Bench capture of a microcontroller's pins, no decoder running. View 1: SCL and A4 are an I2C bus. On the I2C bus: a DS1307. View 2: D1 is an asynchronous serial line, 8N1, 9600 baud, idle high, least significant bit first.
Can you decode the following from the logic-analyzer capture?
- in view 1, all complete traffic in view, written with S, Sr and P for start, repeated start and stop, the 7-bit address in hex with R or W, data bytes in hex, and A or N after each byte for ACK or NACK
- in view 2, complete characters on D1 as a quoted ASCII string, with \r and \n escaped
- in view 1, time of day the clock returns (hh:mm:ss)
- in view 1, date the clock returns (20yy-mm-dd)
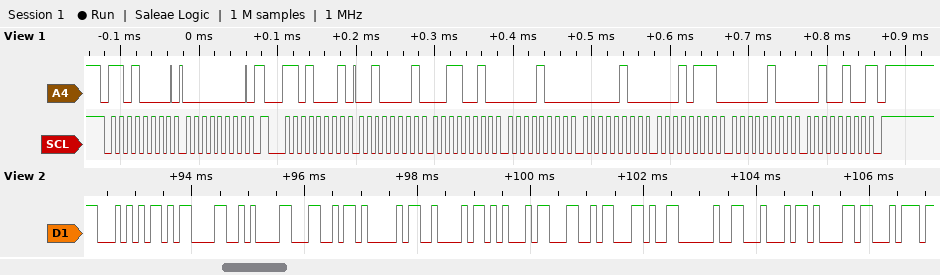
S 68W A 00 A Sr 68R A 21 A 32 A 08 A 04 A 17 A 04 A 24 N P
"T\r\nLABEL, Dat"
08:32:21
2024-04-17
